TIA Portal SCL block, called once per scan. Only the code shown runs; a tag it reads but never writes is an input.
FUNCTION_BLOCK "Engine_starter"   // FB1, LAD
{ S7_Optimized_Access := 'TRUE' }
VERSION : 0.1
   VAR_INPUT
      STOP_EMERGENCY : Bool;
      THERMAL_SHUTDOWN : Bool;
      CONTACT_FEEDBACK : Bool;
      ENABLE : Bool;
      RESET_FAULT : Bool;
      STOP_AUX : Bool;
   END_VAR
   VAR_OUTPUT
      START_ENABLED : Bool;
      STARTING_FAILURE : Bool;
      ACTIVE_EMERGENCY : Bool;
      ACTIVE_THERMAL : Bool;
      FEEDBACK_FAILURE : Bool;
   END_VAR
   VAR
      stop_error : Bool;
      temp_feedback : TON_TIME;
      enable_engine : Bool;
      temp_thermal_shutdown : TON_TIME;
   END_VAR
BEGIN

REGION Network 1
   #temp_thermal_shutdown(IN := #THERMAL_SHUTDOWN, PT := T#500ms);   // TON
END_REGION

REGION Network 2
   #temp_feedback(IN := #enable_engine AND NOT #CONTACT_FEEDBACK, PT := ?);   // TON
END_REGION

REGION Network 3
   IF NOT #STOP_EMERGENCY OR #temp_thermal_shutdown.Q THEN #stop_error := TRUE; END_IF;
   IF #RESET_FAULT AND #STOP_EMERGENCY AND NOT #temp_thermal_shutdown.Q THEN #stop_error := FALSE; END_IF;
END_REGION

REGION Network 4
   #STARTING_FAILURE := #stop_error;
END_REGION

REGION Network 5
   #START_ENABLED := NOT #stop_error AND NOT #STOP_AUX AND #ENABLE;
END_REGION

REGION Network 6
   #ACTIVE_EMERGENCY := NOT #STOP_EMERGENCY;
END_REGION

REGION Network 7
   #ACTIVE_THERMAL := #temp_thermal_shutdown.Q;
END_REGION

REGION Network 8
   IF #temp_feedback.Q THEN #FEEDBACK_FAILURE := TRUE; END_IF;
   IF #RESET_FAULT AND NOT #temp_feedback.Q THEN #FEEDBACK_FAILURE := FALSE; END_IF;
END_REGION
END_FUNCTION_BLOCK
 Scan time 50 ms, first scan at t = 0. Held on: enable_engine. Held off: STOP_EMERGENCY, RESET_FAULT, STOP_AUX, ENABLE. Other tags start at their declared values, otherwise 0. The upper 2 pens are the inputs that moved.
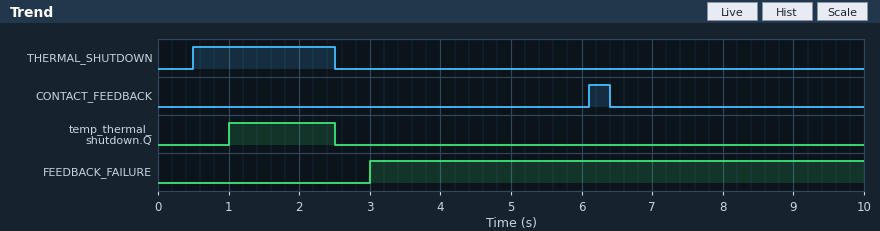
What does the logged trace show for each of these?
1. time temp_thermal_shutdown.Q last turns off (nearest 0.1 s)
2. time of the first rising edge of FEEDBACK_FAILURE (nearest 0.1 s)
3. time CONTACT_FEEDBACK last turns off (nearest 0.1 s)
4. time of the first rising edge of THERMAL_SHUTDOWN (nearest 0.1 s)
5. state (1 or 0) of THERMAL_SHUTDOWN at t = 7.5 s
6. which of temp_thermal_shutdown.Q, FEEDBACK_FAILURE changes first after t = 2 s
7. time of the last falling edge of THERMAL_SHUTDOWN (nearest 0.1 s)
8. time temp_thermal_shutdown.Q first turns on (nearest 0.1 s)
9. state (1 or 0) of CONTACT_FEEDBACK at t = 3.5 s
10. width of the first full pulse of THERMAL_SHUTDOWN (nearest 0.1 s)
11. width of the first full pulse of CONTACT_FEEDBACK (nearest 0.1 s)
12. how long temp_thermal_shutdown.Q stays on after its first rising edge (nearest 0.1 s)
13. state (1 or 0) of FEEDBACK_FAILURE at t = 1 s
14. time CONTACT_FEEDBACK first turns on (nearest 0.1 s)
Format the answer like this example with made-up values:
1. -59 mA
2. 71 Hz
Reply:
1. 2.5 s
2. 3.0 s
3. 6.4 s
4. 0.5 s
5. 0
6. temp_thermal_shutdown.Q
7. 2.5 s
8. 1.0 s
9. 0
10. 2.0 s
11. 0.3 s
12. 1.5 s
13. 0
14. 6.1 s
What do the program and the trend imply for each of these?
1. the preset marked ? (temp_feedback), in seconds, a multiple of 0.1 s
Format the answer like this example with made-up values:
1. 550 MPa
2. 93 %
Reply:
1. 3.0 s
